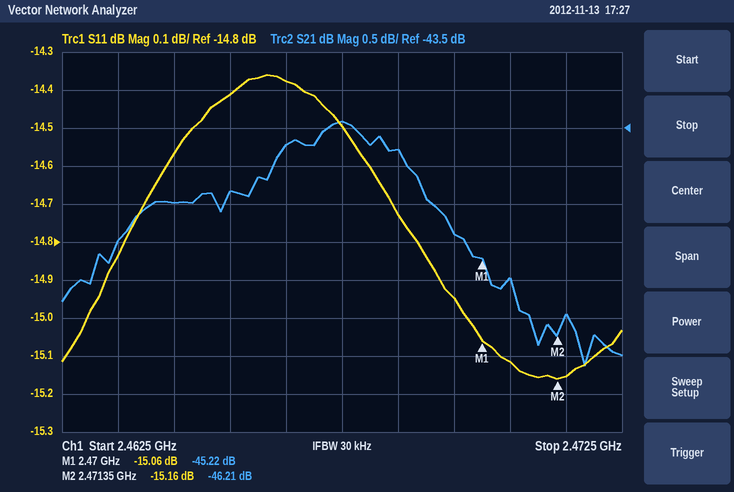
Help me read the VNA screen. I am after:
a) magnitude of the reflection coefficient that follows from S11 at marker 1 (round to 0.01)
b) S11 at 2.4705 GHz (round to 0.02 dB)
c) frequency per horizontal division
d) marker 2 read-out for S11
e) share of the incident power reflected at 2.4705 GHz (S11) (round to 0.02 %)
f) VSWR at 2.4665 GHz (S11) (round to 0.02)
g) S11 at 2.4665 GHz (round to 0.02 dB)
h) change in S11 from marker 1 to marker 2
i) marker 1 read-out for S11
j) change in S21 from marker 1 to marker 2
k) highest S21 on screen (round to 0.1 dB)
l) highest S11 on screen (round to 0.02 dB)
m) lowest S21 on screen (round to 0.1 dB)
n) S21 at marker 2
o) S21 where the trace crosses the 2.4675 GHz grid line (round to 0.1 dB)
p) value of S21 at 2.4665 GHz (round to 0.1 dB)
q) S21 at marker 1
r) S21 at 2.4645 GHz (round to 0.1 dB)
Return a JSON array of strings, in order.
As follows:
["0.18", "-15.12 dB", "1 MHz", "-15.16 dB", "3.08 %", "1.48", "-14.38 dB", "-0.10 dB", "-15.06 dB", "-0.99 dB", "-43.4 dB", "-14.36 dB", "-46.6 dB", "-46.21 dB", "-43.4 dB", "-43.7 dB", "-45.22 dB", "-44.5 dB"]
